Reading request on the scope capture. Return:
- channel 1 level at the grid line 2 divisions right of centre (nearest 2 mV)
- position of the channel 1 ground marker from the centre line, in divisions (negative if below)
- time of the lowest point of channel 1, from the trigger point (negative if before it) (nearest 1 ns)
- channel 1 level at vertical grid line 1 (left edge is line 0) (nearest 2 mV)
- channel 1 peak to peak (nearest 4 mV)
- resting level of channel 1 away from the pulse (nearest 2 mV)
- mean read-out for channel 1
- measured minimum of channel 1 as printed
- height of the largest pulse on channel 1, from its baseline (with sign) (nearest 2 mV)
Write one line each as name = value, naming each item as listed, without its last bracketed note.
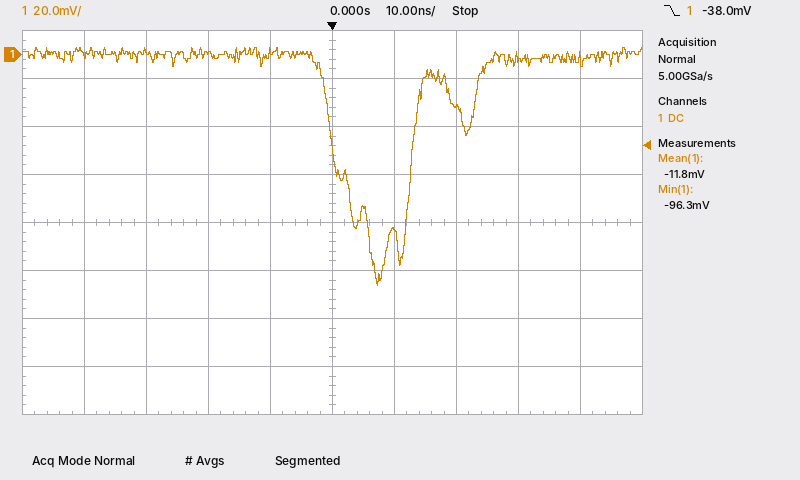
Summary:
channel 1 level at the grid line 2 divisions right of centre = -22 mV
position of the channel 1 ground marker from the centre line, in divisions = +3.5 div
time of the lowest point of channel 1, from the trigger point (negative if before it) = +7 ns
channel 1 level at vertical grid line 1 (left edge is line 0) = 0 mV
channel 1 peak to peak = 100 mV
resting level of channel 1 away from the pulse = 0 mV
mean read-out for channel 1 = -11.8 mV
measured minimum of channel 1 as printed = -96.3 mV
height of the largest pulse on channel 1, from its baseline (with sign) = -96 mV
